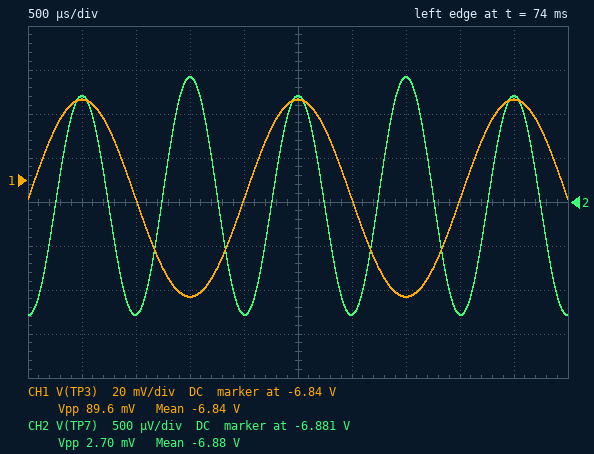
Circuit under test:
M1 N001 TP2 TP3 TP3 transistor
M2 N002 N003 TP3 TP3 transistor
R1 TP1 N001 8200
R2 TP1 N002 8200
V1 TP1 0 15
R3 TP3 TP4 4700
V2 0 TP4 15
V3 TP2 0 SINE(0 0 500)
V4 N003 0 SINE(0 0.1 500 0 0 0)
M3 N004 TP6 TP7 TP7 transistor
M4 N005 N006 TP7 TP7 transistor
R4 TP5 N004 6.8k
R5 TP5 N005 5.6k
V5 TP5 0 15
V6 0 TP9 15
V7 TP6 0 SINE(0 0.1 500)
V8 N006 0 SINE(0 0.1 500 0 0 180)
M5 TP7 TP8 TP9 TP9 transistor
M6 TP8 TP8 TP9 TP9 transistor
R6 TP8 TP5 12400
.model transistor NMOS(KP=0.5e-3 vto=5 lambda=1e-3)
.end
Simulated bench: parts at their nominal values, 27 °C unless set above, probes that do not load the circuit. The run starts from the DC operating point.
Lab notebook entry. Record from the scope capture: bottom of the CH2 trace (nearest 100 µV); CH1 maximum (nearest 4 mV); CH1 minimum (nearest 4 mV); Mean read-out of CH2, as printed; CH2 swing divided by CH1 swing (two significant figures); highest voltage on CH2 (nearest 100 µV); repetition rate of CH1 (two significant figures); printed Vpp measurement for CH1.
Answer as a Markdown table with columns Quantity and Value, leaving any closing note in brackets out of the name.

| Quantity | Value |
|---|---|
| bottom of the CH2 trace | -6.8828 V |
| CH1 maximum | -6.804 V |
| CH1 minimum | -6.892 V |
| Mean read-out of CH2, as printed | -6.88 V |
| CH2 swing divided by CH1 swing | 0.030 |
| highest voltage on CH2 | -6.8801 V |
| repetition rate of CH1 | 500 Hz |
| printed Vpp measurement for CH1 | 89.6 mV |
